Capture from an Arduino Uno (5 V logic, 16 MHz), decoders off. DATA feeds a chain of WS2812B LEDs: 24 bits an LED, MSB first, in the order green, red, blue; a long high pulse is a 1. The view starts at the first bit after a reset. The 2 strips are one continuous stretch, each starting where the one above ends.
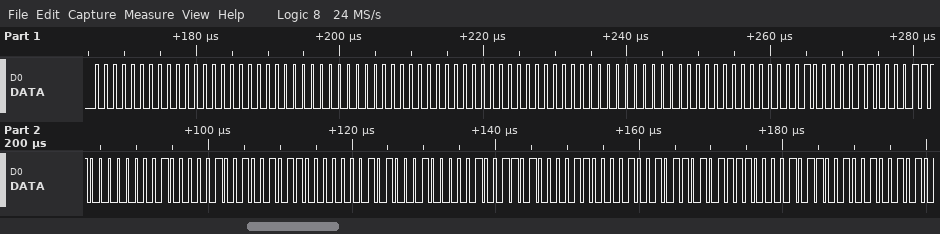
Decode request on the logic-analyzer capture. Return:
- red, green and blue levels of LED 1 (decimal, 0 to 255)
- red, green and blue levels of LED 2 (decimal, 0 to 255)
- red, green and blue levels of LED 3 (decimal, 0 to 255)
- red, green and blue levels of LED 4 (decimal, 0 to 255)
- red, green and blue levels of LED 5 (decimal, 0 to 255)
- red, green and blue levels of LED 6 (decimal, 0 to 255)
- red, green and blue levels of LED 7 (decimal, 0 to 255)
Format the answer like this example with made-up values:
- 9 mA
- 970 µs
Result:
- 0, 0, 0
- 0, 0, 0
- 0, 0, 0
- 6, 1, 28
- 9, 2, 44
- 16, 5, 77
- 37, 12, 175
